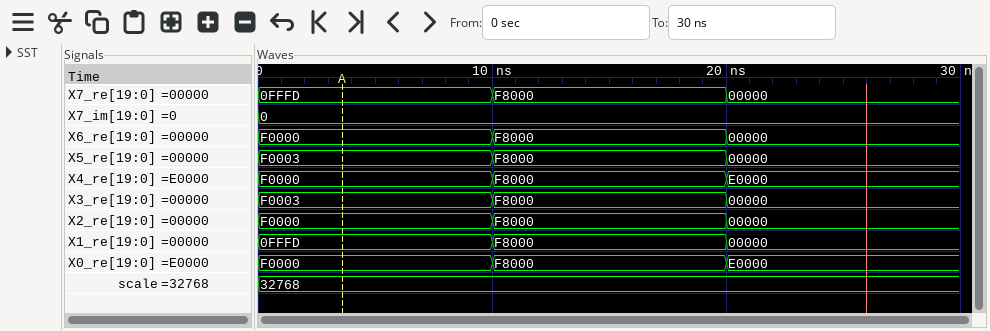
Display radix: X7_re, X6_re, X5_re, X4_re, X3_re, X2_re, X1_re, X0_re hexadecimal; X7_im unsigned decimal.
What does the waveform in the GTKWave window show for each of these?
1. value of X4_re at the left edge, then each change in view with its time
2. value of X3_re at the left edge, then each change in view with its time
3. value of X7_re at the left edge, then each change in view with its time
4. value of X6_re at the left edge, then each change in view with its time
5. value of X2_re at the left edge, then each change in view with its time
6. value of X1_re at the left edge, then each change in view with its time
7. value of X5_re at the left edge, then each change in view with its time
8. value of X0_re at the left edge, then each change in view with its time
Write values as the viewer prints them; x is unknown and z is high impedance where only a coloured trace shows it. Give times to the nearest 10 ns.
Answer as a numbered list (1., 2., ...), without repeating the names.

1. F0000, F8000 at 10 ns, E0000 at 20 ns
2. F0003, F8000 at 10 ns, 00000 at 20 ns
3. 0FFFD, F8000 at 10 ns, 00000 at 20 ns
4. F0000, F8000 at 10 ns, 00000 at 20 ns
5. F0000, F8000 at 10 ns, 00000 at 20 ns
6. 0FFFD, F8000 at 10 ns, 00000 at 20 ns
7. F0003, F8000 at 10 ns, 00000 at 20 ns
8. F0000, F8000 at 10 ns, E0000 at 20 ns
